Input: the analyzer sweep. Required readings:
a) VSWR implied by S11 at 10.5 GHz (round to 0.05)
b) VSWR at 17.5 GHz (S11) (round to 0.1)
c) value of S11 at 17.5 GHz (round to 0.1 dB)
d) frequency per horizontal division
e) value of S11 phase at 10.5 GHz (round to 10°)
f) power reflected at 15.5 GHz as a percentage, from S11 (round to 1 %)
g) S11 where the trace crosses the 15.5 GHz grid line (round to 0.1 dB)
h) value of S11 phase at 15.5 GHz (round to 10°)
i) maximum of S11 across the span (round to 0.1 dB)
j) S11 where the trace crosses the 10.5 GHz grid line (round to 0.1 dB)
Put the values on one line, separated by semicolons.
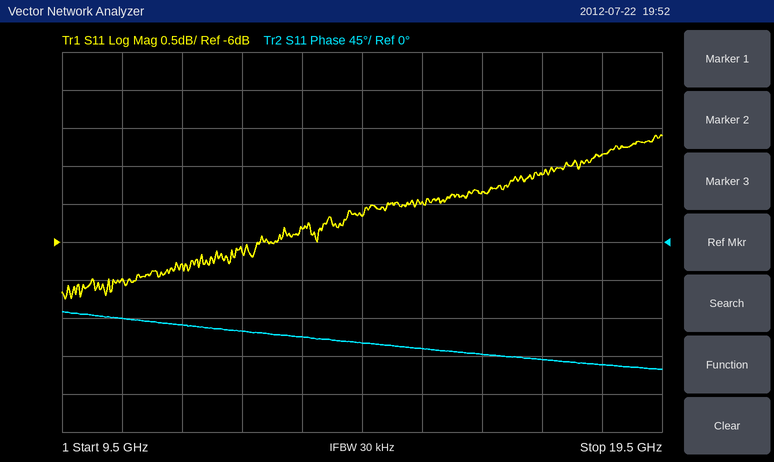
2.80; 3.5; -5.1 dB; 1 GHz; -90°; 28 %; -5.5 dB; -130°; -4.6 dB; -6.5 dB
